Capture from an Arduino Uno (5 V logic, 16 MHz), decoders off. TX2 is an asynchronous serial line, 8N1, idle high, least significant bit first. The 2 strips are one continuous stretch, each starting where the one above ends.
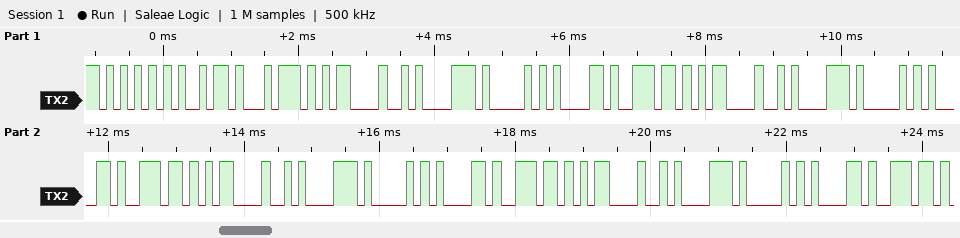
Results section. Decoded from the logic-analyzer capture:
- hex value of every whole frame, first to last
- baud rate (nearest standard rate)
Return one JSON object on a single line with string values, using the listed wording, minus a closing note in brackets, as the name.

{"hex value of every whole frame, first to last": "55 69 74 0D 0A 41 61 6E 0D 0A 41 61 6E 0D 0A 41 61 6E 0D 0A 41 61 6E", "baud rate": "9600 baud"}
